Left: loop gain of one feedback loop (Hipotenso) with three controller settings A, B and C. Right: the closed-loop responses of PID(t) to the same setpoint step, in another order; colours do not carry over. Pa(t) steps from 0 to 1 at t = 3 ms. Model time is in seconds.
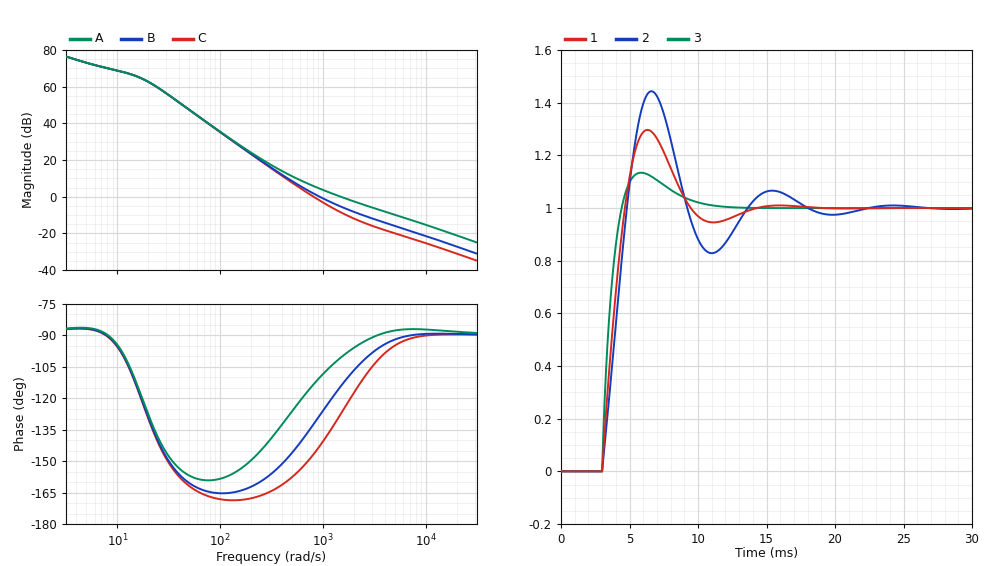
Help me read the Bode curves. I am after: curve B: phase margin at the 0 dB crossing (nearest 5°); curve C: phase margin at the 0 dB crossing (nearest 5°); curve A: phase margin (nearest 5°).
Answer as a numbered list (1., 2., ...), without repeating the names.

1. 50°
2. 35°
3. 80°
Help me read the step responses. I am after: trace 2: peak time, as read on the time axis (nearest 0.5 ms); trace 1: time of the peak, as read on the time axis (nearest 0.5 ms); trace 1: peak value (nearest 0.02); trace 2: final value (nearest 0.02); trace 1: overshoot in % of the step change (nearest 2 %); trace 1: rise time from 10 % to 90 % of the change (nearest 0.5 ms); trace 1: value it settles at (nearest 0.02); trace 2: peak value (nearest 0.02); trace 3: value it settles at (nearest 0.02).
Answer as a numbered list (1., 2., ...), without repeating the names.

1. 6.5 ms
2. 6.5 ms
3. 1.30
4. 1.00
5. 30 %
6. 1.5 ms
7. 1.00
8. 1.44
9. 1.00
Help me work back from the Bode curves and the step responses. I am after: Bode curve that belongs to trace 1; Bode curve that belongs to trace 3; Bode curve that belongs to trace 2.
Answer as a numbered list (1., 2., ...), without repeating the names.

1. B
2. A
3. C
